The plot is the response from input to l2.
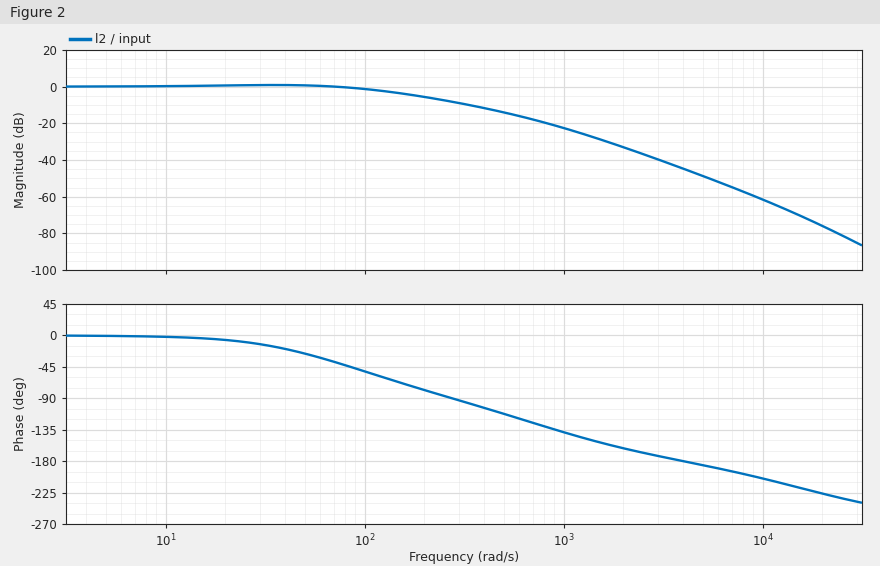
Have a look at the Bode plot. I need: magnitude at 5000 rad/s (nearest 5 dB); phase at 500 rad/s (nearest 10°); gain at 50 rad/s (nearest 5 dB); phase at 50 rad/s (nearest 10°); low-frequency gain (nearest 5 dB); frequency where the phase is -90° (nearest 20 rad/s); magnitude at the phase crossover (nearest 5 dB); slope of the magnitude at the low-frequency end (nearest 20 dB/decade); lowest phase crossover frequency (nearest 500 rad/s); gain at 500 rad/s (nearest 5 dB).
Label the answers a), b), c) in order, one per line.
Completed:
a) -50 dB
b) -110°
c) 0 dB
d) -30°
e) 0 dB
f) 280 rad/s
g) -45 dB
h) 0 dB/decade
i) 4000 rad/s
j) -15 dB
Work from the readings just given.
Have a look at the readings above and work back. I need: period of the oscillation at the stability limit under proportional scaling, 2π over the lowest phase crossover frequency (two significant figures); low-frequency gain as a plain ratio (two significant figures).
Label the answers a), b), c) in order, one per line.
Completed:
a) 0.0016 s
b) 1.0
